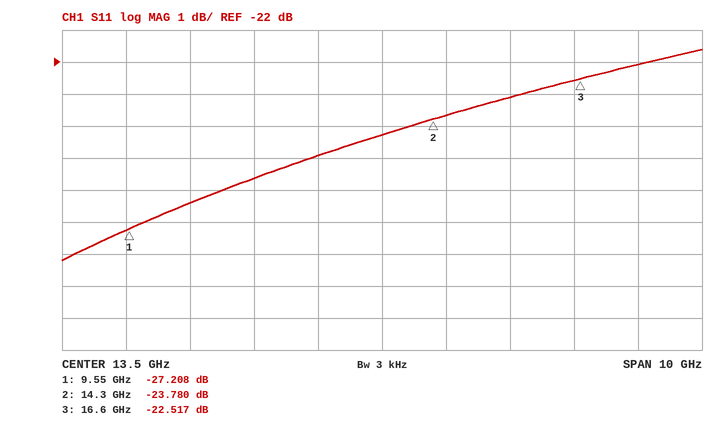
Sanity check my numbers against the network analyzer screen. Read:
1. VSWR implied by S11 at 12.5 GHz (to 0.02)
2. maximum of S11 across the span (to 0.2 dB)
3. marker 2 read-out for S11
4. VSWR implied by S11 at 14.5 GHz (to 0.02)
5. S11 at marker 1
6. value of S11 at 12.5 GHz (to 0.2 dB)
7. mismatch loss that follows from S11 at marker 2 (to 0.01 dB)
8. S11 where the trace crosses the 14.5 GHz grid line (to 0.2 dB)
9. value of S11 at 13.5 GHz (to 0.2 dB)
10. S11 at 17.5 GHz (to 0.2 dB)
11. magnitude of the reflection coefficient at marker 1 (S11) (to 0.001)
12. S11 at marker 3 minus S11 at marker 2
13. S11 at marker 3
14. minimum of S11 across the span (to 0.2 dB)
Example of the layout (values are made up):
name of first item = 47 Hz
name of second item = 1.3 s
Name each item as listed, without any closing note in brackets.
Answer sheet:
VSWR implied by S11 at 12.5 GHz = 1.12
maximum of S11 across the span = -21.6 dB
marker 2 read-out for S11 = -23.780 dB
VSWR implied by S11 at 14.5 GHz = 1.14
S11 at marker 1 = -27.208 dB
value of S11 at 12.5 GHz = -25.0 dB
mismatch loss that follows from S11 at marker 2 = 0.02 dB
S11 where the trace crosses the 14.5 GHz grid line = -23.6 dB
value of S11 at 13.5 GHz = -24.2 dB
S11 at 17.5 GHz = -22.0 dB
magnitude of the reflection coefficient at marker 1 (S11) = 0.044
S11 at marker 3 minus S11 at marker 2 = 1.263 dB
S11 at marker 3 = -22.517 dB
minimum of S11 across the span = -28.2 dB
